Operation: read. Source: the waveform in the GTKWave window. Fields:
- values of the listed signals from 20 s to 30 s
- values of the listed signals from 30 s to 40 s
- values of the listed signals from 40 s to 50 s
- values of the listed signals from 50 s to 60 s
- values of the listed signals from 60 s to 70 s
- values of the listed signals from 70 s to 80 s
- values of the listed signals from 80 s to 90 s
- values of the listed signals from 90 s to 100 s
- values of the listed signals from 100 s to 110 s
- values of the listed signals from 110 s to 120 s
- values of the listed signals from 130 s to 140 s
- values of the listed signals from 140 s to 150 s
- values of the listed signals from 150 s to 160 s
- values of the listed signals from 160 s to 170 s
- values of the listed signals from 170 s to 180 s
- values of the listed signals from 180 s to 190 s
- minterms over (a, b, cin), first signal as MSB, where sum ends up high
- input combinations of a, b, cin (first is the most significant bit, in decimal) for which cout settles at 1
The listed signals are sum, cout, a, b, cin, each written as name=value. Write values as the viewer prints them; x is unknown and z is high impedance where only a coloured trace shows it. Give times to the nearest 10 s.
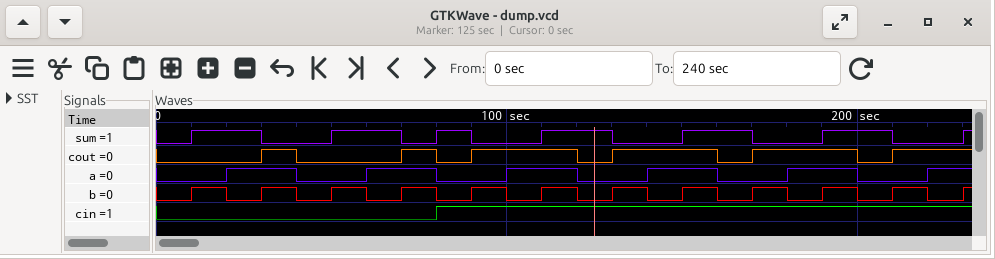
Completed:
sum=1, cout=0, a=1, b=0, cin=0
sum=0, cout=1, a=1, b=1, cin=0
sum=0, cout=0, a=0, b=0, cin=0
sum=1, cout=0, a=0, b=1, cin=0
sum=1, cout=0, a=1, b=0, cin=0
sum=0, cout=1, a=1, b=1, cin=0
sum=1, cout=0, a=0, b=0, cin=1
sum=0, cout=1, a=0, b=1, cin=1
sum=0, cout=1, a=1, b=0, cin=1
sum=1, cout=1, a=1, b=1, cin=1
sum=0, cout=1, a=0, b=1, cin=1
sum=0, cout=1, a=1, b=0, cin=1
sum=1, cout=1, a=1, b=1, cin=1
sum=1, cout=0, a=0, b=0, cin=1
sum=0, cout=1, a=0, b=1, cin=1
sum=0, cout=1, a=1, b=0, cin=1
1, 2, 4, 7
3, 5, 6, 7
